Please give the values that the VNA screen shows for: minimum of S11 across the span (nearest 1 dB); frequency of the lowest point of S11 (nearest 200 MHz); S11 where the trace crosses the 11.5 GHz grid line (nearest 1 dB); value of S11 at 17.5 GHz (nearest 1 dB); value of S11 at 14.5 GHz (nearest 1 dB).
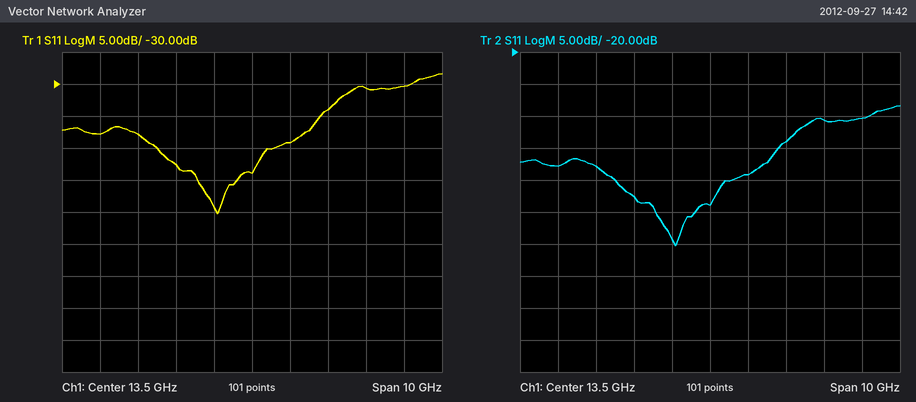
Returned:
-50 dB
12.6 GHz
-43 dB
-30 dB
-39 dB
